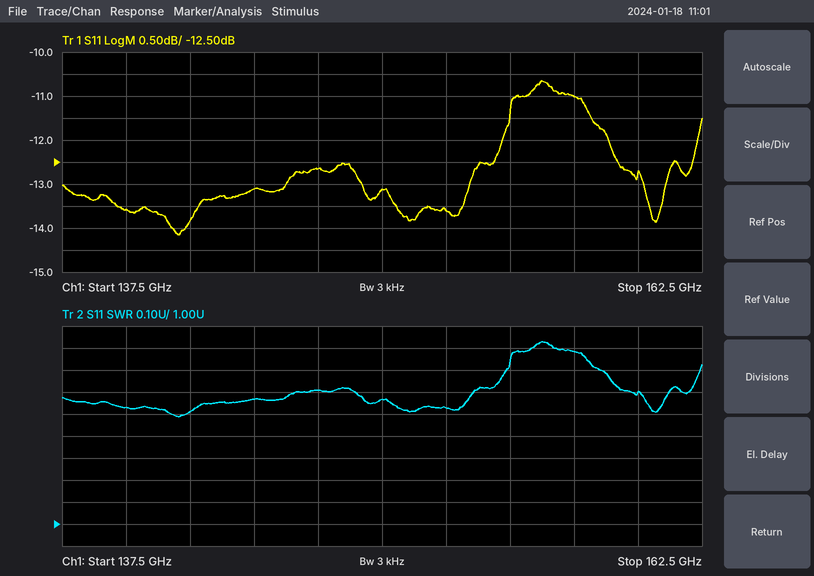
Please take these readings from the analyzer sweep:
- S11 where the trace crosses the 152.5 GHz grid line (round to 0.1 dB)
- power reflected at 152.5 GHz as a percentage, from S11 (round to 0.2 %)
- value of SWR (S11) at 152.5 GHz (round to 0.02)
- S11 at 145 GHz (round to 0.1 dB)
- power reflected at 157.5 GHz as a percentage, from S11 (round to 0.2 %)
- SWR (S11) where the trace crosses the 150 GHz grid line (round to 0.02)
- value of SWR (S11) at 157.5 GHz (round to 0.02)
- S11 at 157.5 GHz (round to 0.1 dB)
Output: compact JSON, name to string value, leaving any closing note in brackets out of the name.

{"S11 where the trace crosses the 152.5 GHz grid line": "-13.6 dB", "power reflected at 152.5 GHz as a percentage, from S11": "4.4 %", "value of SWR (S11) at 152.5 GHz": "1.52", "S11 at 145 GHz": "-13.1 dB", "power reflected at 157.5 GHz as a percentage, from S11": "8.0 %", "SWR (S11) where the trace crosses the 150 GHz grid line": "1.56", "value of SWR (S11) at 157.5 GHz": "1.78", "S11 at 157.5 GHz": "-11.0 dB"}
